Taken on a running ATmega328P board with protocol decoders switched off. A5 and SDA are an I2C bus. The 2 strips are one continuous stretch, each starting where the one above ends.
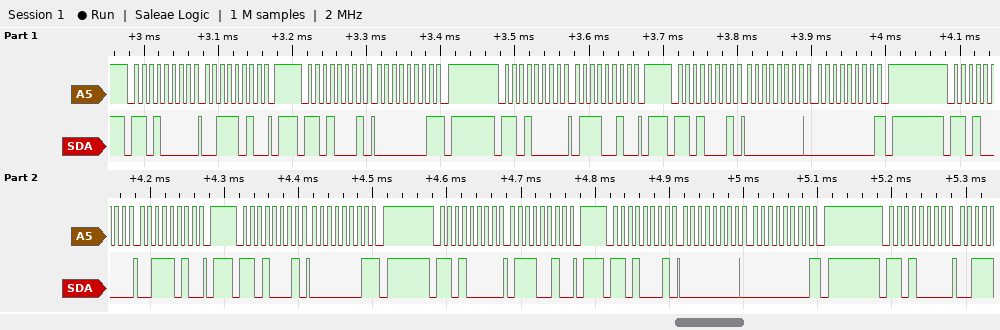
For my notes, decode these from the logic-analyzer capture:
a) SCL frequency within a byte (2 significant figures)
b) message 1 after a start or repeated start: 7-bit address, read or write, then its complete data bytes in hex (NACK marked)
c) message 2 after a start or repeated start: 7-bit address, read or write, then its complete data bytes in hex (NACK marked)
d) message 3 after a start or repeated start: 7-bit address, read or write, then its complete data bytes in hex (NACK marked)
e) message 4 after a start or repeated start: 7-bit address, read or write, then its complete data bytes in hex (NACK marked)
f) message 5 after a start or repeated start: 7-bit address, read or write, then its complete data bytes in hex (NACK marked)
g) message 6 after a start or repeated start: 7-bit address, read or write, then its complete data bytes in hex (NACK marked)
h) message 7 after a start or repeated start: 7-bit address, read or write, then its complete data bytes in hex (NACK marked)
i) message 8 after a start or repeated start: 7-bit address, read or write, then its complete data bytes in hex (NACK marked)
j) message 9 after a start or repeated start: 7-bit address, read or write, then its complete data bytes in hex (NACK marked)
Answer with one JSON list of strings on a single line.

["100 kHz", "0x68 write: 3A", "0x68 read: 01 NACK", "0x68 write: 72", "0x68 read: 00 00 NACK", "0x68 write: 3A", "0x68 read: 01 NACK", "0x68 write: 72", "0x68 read: 00 00 NACK", "0x68 write"]
